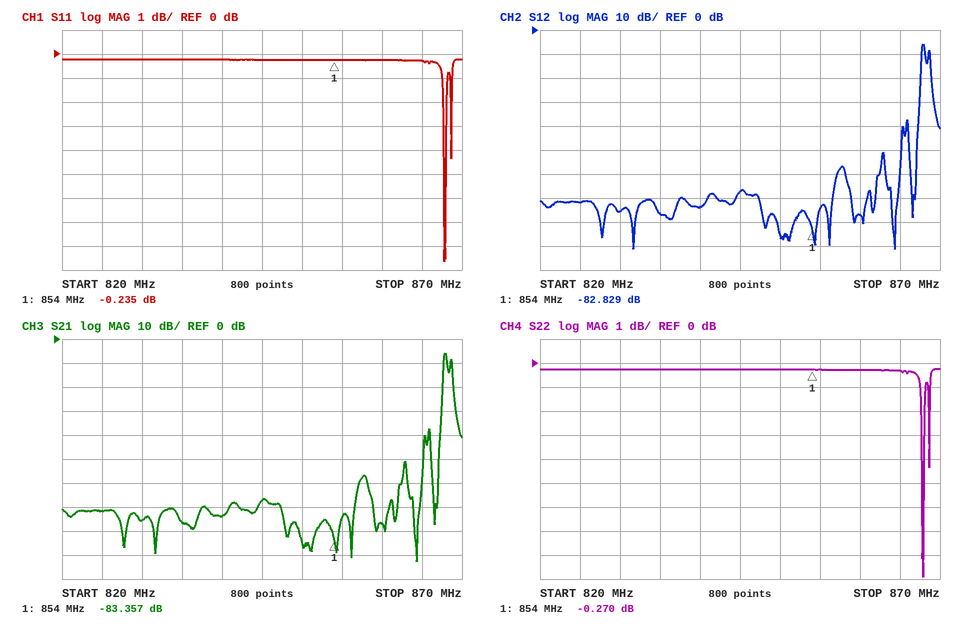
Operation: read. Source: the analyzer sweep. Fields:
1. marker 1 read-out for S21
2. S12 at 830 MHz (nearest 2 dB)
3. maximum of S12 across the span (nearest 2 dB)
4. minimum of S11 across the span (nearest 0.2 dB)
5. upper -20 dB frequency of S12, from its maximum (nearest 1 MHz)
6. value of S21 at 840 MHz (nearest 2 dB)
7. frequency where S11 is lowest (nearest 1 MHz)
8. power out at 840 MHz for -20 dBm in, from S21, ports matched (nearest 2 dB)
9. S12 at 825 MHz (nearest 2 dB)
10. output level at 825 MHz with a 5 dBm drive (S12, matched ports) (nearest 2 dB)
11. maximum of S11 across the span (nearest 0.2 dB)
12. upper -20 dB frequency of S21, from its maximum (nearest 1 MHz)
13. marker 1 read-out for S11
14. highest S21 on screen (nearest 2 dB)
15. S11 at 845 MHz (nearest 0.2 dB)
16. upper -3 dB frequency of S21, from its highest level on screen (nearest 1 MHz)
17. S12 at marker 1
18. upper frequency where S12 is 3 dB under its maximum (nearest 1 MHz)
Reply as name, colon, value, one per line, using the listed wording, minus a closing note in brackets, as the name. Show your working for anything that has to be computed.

marker 1 read-out for S21: -83.357 dB
S12 at 830 MHz: -76 dB
maximum of S12 across the span: -6 dB
minimum of S11 across the span: -8.6 dB
upper -20 dB frequency of S12, from its maximum: 869 MHz
value of S21 at 840 MHz: -74 dB
frequency where S11 is lowest: 868 MHz
power out at 840 MHz for -20 dBm in, from S21, ports matched: -20 dBm + (-74 dB) = -94 dBm
S12 at 825 MHz: -72 dB
output level at 825 MHz with a 5 dBm drive (S12, matched ports): 5 dBm + (-72 dB) = -66 dBm
maximum of S11 across the span: -0.2 dB
upper -20 dB frequency of S21, from its maximum: 869 MHz
marker 1 read-out for S11: -0.235 dB
highest S21 on screen: -6 dB
S11 at 845 MHz: -0.2 dB
upper -3 dB frequency of S21, from its highest level on screen: 868 MHz
S12 at marker 1: -82.829 dB
upper frequency where S12 is 3 dB under its maximum: 868 MHz
